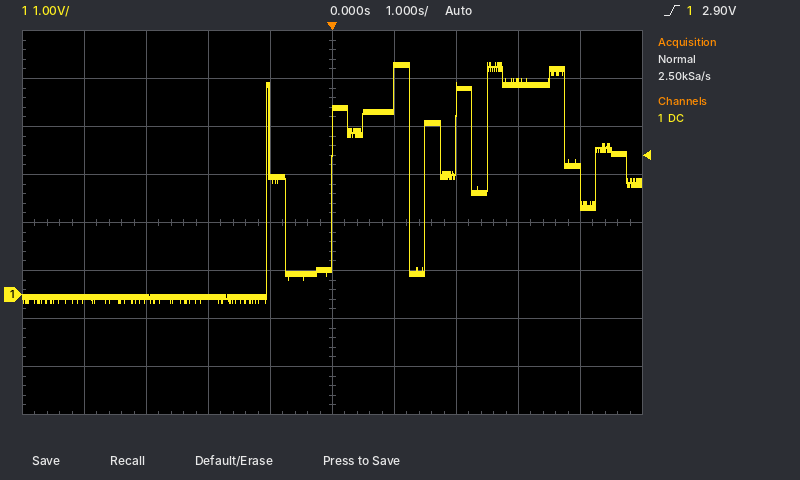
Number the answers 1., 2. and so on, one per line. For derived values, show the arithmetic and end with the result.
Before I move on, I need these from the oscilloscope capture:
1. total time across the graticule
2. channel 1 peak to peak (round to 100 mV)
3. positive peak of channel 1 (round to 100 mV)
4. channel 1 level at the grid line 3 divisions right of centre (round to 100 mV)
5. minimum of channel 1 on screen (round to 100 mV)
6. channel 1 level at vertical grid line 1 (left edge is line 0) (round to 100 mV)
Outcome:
1. 10 s
2. 4.8 V − (-200 mV) = 5.0 V
3. 4.8 V
4. 4.4 V
5. -200 mV
6. -100 mV
